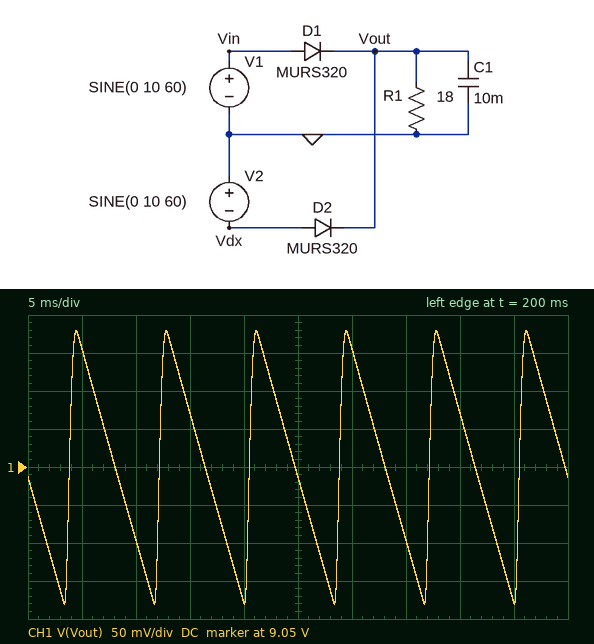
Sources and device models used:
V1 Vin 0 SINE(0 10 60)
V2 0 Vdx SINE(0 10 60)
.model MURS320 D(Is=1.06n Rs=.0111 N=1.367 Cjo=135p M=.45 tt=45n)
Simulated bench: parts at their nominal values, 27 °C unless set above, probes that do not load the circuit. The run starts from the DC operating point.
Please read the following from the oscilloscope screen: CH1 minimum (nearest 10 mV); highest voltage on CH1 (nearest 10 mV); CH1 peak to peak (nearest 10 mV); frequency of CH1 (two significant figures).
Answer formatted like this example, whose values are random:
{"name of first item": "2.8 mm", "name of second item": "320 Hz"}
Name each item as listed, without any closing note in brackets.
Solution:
{"CH1 minimum": "8.87 V", "highest voltage on CH1": "9.23 V", "CH1 peak to peak": "360 mV", "frequency of CH1": "120 Hz"}
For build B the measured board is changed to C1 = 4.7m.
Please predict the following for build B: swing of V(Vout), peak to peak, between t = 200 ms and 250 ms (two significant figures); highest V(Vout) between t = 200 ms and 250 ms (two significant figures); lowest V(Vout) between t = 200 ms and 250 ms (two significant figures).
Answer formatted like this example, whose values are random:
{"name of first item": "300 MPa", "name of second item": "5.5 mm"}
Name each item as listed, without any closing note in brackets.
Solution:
{"swing of V(Vout), peak to peak, between t = 200 ms and 250 ms": "730 mV", "highest V(Vout) between t = 200 ms and 250 ms": "9.3 V", "lowest V(Vout) between t = 200 ms and 250 ms": "8.5 V"}
